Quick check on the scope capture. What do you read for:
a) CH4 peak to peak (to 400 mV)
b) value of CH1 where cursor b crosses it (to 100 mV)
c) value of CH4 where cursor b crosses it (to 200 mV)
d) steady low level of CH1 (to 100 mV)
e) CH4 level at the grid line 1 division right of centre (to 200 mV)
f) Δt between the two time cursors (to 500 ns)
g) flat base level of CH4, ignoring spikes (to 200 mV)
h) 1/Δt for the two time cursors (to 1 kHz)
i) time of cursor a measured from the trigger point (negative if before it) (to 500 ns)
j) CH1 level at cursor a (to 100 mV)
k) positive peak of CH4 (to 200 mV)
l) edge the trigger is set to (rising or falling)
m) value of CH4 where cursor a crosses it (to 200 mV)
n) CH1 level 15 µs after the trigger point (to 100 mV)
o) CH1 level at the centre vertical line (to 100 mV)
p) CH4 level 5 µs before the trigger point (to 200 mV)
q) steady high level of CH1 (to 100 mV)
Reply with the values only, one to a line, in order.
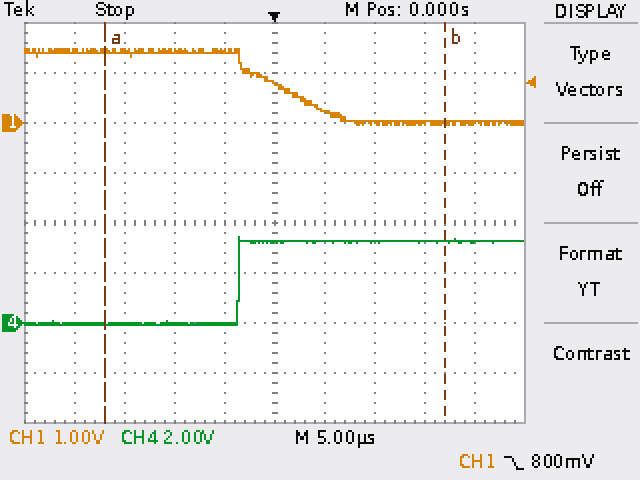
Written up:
3.6 V
0.0 V
3.2 V
0.0 V
3.2 V
34.0 µs
0.0 V
29 kHz
-17.0 µs
1.4 V
3.4 V
falling
0.0 V
0.0 V
800 mV
0.0 V
1.4 V
